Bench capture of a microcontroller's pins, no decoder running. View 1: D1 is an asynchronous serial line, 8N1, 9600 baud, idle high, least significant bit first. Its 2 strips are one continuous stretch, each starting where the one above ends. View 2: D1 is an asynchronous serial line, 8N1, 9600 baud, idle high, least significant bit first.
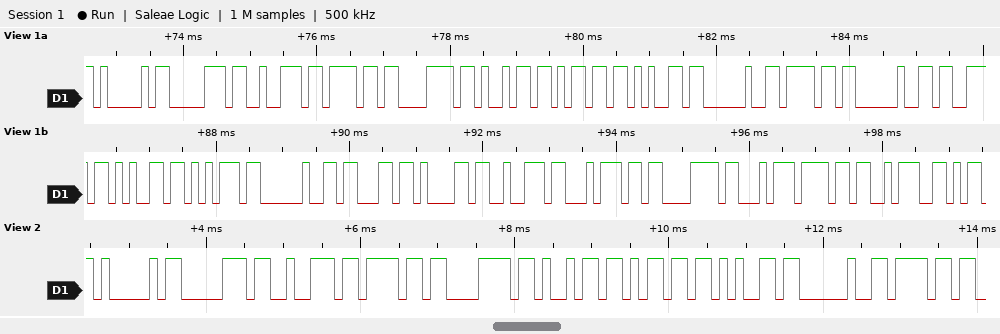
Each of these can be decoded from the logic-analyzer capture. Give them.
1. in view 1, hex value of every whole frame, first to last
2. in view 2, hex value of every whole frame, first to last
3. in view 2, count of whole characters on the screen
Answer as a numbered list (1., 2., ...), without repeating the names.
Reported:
1. 41 70 72 6F 78 69 6D 65 20 6F 20 73 65 75 20 63 61 72 74 C3 A3 6F 3A
2. 41 70 72 6F 78 69 6D 65 20 6F
3. 10
